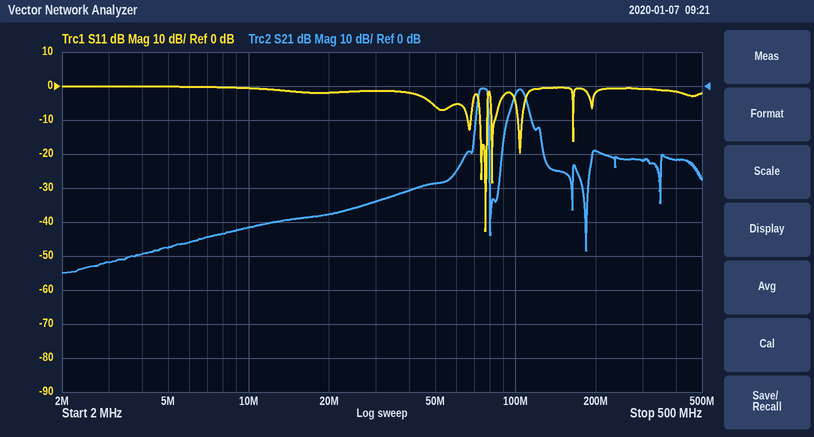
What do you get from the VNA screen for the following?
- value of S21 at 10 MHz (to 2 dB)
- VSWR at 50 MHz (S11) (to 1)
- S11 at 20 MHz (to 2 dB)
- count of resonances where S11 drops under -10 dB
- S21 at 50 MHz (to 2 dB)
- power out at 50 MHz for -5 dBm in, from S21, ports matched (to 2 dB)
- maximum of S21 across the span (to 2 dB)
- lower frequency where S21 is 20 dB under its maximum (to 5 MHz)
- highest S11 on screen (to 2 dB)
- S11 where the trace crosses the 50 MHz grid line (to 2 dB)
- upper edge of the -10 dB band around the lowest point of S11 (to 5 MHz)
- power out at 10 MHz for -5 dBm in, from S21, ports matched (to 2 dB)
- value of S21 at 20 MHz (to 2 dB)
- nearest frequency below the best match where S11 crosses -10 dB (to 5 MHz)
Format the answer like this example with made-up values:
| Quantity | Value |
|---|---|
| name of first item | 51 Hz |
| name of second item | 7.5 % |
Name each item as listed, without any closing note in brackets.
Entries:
| Quantity | Value |
|---|---|
| value of S21 at 10 MHz | -42 dB |
| VSWR at 50 MHz (S11) | 3 |
| S11 at 20 MHz | -2 dB |
| count of resonances where S11 drops under -10 dB | 6 |
| S21 at 50 MHz | -28 dB |
| power out at 50 MHz for -5 dBm in, from S21, ports matched | -34 dBm |
| maximum of S21 across the span | 0 dB |
| lower frequency where S21 is 20 dB under its maximum | 65 MHz |
| highest S11 on screen | 0 dB |
| S11 where the trace crosses the 50 MHz grid line | -6 dB |
| upper edge of the -10 dB band around the lowest point of S11 | 80 MHz |
| power out at 10 MHz for -5 dBm in, from S21, ports matched | -46 dBm |
| value of S21 at 20 MHz | -38 dB |
| nearest frequency below the best match where S11 crosses -10 dB | 75 MHz |
